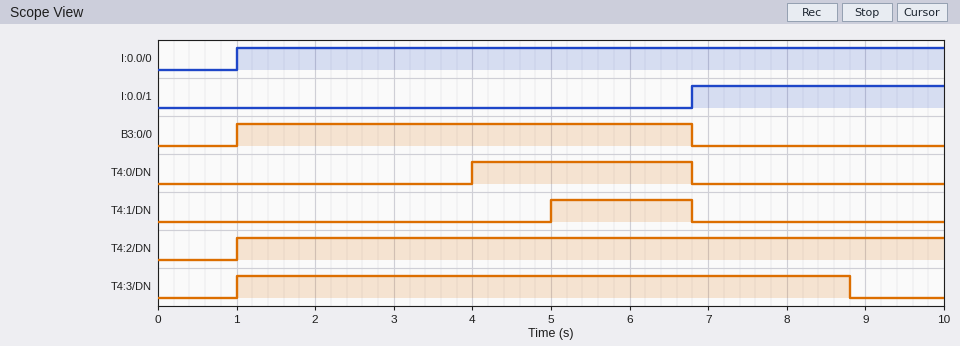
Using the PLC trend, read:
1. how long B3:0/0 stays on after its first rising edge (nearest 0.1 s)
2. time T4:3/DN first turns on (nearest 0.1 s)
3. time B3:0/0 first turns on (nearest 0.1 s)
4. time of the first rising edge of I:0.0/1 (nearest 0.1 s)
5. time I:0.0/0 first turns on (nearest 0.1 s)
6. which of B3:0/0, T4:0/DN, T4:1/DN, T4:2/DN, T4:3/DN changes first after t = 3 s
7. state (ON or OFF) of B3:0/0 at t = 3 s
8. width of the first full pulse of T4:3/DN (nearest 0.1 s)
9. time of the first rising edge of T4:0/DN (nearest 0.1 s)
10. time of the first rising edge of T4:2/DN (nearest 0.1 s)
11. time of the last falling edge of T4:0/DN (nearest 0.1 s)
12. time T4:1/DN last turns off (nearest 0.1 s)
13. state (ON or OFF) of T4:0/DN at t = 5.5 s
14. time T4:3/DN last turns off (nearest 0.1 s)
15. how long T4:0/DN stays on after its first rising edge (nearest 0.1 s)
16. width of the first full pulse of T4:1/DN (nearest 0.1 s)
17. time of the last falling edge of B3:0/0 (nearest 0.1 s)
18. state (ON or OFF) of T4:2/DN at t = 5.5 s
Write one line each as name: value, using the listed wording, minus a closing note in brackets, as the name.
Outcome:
how long B3:0/0 stays on after its first rising edge: 5.8 s
time T4:3/DN first turns on: 1.0 s
time B3:0/0 first turns on: 1.0 s
time of the first rising edge of I:0.0/1: 6.8 s
time I:0.0/0 first turns on: 1.0 s
which of B3:0/0, T4:0/DN, T4:1/DN, T4:2/DN, T4:3/DN changes first after t = 3 s: T4:0/DN
state (ON or OFF) of B3:0/0 at t = 3 s: ON
width of the first full pulse of T4:3/DN: 7.8 s
time of the first rising edge of T4:0/DN: 4.0 s
time of the first rising edge of T4:2/DN: 1.0 s
time of the last falling edge of T4:0/DN: 6.8 s
time T4:1/DN last turns off: 6.8 s
state (ON or OFF) of T4:0/DN at t = 5.5 s: ON
time T4:3/DN last turns off: 8.8 s
how long T4:0/DN stays on after its first rising edge: 2.8 s
width of the first full pulse of T4:1/DN: 1.8 s
time of the last falling edge of B3:0/0: 6.8 s
state (ON or OFF) of T4:2/DN at t = 5.5 s: ON
